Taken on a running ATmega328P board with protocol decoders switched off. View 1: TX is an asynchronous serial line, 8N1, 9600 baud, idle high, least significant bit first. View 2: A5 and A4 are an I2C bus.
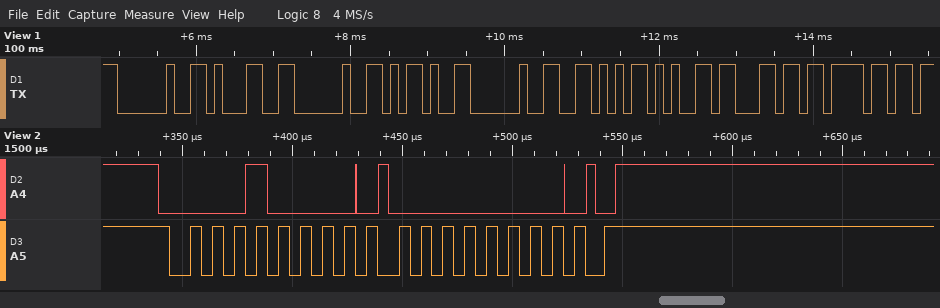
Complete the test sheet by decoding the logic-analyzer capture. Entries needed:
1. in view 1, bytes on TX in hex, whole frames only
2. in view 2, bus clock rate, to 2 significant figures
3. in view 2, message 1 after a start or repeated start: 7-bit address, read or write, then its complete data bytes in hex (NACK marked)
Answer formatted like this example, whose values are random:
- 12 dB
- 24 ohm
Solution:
- 20 31 20 2D 20 56 65 6C 6F
- 100 kHz
- 0x08 write: 00
